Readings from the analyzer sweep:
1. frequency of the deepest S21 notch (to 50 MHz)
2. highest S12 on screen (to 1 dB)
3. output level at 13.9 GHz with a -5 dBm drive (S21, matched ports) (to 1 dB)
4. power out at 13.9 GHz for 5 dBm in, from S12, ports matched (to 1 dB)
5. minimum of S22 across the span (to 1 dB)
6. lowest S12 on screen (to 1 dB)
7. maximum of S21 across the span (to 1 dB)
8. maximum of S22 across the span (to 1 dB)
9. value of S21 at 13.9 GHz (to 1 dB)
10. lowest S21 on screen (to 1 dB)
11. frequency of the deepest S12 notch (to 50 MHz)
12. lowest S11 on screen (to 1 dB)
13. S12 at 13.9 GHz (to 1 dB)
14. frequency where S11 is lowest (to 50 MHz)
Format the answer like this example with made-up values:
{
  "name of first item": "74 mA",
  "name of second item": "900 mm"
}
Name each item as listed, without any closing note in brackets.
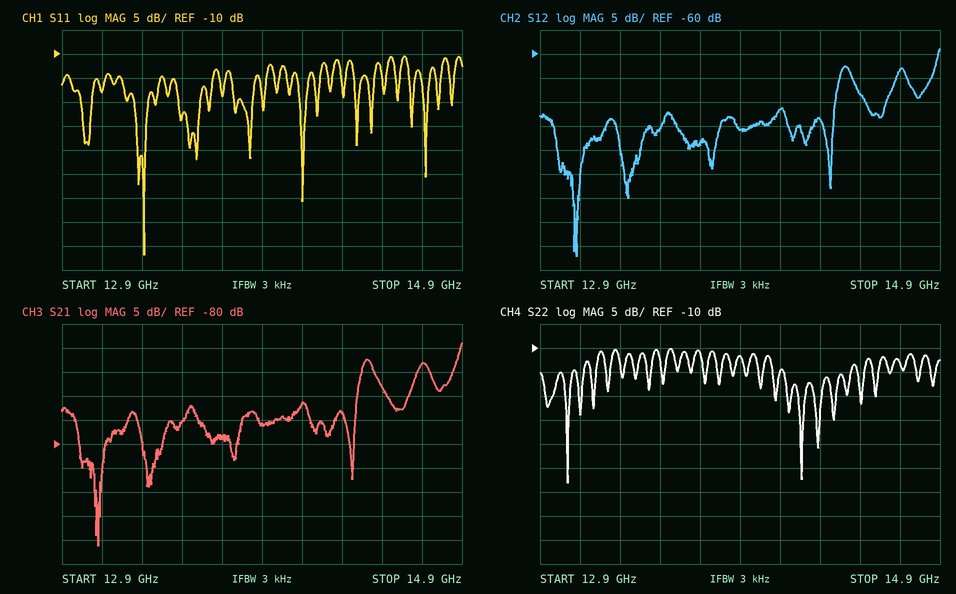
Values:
{
  "frequency of the deepest S21 notch": "13.10 GHz",
  "highest S12 on screen": "-59 dB",
  "output level at 13.9 GHz with a -5 dBm drive (S21, matched ports)": "-81 dBm",
  "power out at 13.9 GHz for 5 dBm in, from S12, ports matched": "-71 dBm",
  "minimum of S22 across the span": "-38 dB",
  "lowest S12 on screen": "-102 dB",
  "maximum of S21 across the span": "-59 dB",
  "maximum of S22 across the span": "-10 dB",
  "value of S21 at 13.9 GHz": "-76 dB",
  "lowest S21 on screen": "-101 dB",
  "frequency of the deepest S12 notch": "13.10 GHz",
  "lowest S11 on screen": "-52 dB",
  "S12 at 13.9 GHz": "-76 dB",
  "frequency where S11 is lowest": "13.30 GHz"
}
